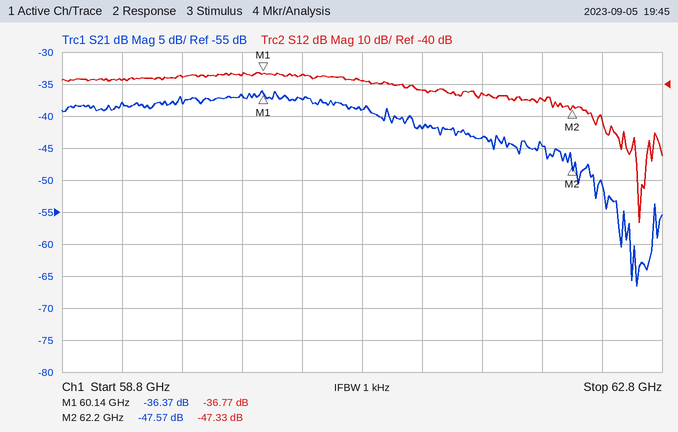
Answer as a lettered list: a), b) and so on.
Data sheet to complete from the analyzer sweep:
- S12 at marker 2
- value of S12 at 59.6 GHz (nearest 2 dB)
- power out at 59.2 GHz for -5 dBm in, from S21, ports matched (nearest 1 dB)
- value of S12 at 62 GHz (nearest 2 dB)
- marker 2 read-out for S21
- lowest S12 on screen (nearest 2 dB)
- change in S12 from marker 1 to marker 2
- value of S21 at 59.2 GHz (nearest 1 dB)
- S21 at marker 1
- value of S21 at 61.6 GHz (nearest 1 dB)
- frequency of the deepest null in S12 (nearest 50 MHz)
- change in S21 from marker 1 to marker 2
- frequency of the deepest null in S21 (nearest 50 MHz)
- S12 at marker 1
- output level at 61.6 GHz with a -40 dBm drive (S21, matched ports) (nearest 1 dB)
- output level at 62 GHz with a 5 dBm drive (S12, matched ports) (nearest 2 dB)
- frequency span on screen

a) -47.33 dB
b) -38 dB
c) -43 dBm
d) -44 dB
e) -47.57 dB
f) -84 dB
g) -10.56 dB
h) -38 dB
i) -36.37 dB
j) -43 dB
k) 62.65 GHz
l) -11.20 dB
m) 62.65 GHz
n) -36.77 dB
o) -83 dBm
p) -40 dBm
q) 4 GHz
